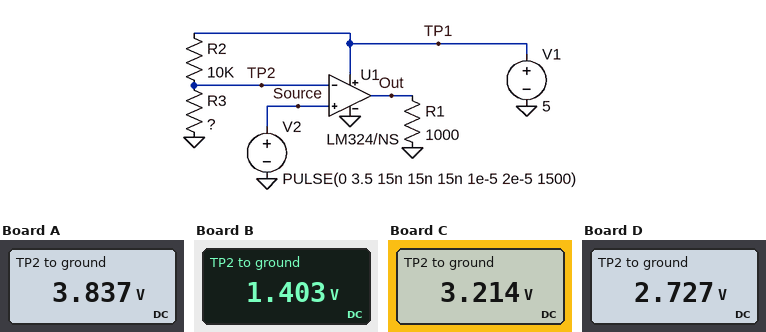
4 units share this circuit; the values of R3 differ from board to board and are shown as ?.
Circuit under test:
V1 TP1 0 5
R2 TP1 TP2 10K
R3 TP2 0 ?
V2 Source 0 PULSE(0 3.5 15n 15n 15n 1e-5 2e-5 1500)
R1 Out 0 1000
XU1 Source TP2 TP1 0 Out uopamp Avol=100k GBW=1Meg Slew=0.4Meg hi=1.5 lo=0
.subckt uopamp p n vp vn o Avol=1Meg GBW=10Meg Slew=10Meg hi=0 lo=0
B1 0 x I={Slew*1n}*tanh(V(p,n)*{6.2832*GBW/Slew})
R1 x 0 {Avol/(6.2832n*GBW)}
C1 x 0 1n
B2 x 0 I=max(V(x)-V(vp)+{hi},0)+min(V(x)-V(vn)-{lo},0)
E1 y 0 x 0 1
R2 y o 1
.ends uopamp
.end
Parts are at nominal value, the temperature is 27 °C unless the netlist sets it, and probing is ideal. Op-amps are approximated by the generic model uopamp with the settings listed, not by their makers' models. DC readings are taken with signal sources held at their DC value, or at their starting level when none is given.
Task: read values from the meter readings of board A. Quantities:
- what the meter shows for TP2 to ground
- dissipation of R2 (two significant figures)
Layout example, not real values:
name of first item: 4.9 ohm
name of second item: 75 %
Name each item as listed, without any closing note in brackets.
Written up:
what the meter shows for TP2 to ground: 3.837 V
dissipation of R2: 140 µW
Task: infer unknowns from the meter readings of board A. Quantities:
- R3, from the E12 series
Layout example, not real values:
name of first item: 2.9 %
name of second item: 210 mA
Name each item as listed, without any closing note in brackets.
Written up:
R3, from the E12 series: 33 kΩ
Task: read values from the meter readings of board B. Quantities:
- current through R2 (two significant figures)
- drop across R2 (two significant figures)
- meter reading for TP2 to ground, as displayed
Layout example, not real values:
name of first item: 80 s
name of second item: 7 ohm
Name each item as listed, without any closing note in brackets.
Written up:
current through R2: 360 µA
drop across R2: 3.6 V
meter reading for TP2 to ground, as displayed: 1.403 V
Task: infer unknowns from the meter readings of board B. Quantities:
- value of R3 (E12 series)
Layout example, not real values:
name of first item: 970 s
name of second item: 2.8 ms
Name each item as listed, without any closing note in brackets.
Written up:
value of R3: 3.9 kΩ
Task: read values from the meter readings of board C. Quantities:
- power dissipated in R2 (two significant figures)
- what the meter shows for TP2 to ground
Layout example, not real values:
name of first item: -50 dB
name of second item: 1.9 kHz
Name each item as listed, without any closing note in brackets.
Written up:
power dissipated in R2: 320 µW
what the meter shows for TP2 to ground: 3.214 V
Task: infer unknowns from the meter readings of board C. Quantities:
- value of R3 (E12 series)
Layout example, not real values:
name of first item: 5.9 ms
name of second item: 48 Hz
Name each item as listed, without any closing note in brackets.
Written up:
value of R3: 18 kΩ
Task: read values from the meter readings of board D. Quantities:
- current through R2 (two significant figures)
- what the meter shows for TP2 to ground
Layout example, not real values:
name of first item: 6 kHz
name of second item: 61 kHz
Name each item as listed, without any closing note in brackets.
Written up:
current through R2: 230 µA
what the meter shows for TP2 to ground: 2.727 V
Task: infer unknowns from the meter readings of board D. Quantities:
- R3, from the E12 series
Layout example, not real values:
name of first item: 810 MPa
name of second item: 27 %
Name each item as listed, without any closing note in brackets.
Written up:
R3, from the E12 series: 12 kΩ
